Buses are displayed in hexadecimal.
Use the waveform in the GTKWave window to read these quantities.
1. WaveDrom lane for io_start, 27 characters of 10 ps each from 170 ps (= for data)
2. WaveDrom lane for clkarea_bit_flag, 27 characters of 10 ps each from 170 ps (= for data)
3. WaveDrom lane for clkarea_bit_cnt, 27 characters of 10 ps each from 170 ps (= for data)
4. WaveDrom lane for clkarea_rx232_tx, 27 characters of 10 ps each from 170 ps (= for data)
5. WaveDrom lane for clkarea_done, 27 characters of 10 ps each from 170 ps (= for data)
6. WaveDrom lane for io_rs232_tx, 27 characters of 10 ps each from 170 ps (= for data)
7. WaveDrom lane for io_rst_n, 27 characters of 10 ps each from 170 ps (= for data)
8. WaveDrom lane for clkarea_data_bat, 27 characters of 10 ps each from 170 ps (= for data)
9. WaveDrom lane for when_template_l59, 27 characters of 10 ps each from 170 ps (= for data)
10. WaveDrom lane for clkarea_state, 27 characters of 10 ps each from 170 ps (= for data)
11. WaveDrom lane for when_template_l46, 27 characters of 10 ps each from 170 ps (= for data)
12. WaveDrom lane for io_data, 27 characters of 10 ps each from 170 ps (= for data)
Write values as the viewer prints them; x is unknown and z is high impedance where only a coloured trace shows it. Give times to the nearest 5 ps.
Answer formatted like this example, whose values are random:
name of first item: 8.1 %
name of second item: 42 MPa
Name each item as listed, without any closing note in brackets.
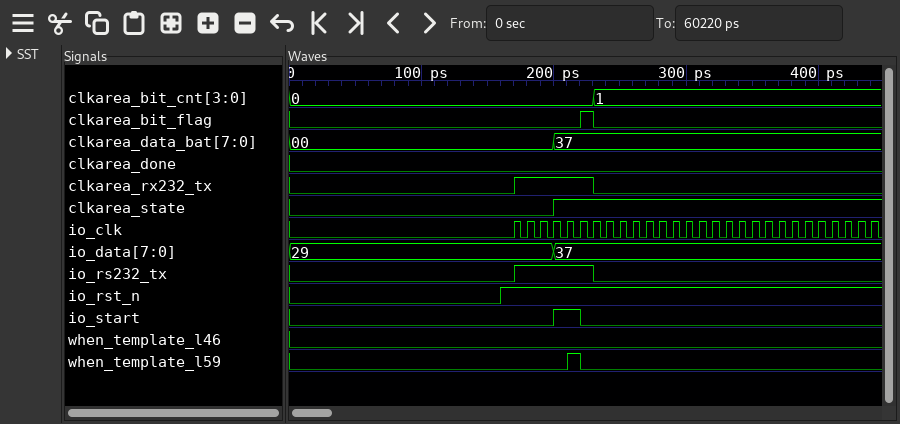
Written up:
WaveDrom lane for io_start, 27 characters of 10 ps each from 170 ps: {name: 'io_start', wave: '0..1.0.....................'}
WaveDrom lane for clkarea_bit_flag, 27 characters of 10 ps each from 170 ps: {name: 'clkarea_bit_flag', wave: '0....10....................'}
WaveDrom lane for clkarea_bit_cnt, 27 characters of 10 ps each from 170 ps: {name: 'clkarea_bit_cnt', wave: '=.....=....................', data: '0 1'}
WaveDrom lane for clkarea_rx232_tx, 27 characters of 10 ps each from 170 ps: {name: 'clkarea_rx232_tx', wave: '1.....0....................'}
WaveDrom lane for clkarea_done, 27 characters of 10 ps each from 170 ps: {name: 'clkarea_done', wave: '0..........................'}
WaveDrom lane for io_rs232_tx, 27 characters of 10 ps each from 170 ps: {name: 'io_rs232_tx', wave: '1.....0....................'}
WaveDrom lane for io_rst_n, 27 characters of 10 ps each from 170 ps: {name: 'io_rst_n', wave: '1..........................'}
WaveDrom lane for clkarea_data_bat, 27 characters of 10 ps each from 170 ps: {name: 'clkarea_data_bat', wave: '=..=.......................', data: '00 37'}
WaveDrom lane for when_template_l59, 27 characters of 10 ps each from 170 ps: {name: 'when_template_l59', wave: '0...10.....................'}
WaveDrom lane for clkarea_state, 27 characters of 10 ps each from 170 ps: {name: 'clkarea_state', wave: '0..1.......................'}
WaveDrom lane for when_template_l46, 27 characters of 10 ps each from 170 ps: {name: 'when_template_l46', wave: '0..........................'}
WaveDrom lane for io_data, 27 characters of 10 ps each from 170 ps: {name: 'io_data', wave: '=..=.......................', data: '29 37'}
